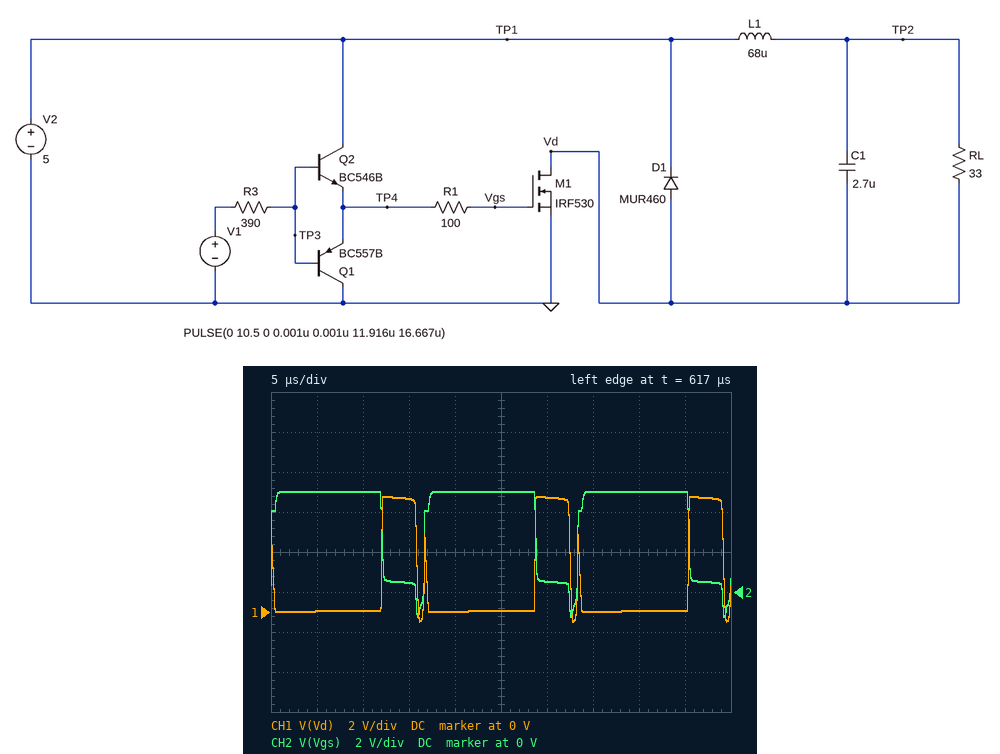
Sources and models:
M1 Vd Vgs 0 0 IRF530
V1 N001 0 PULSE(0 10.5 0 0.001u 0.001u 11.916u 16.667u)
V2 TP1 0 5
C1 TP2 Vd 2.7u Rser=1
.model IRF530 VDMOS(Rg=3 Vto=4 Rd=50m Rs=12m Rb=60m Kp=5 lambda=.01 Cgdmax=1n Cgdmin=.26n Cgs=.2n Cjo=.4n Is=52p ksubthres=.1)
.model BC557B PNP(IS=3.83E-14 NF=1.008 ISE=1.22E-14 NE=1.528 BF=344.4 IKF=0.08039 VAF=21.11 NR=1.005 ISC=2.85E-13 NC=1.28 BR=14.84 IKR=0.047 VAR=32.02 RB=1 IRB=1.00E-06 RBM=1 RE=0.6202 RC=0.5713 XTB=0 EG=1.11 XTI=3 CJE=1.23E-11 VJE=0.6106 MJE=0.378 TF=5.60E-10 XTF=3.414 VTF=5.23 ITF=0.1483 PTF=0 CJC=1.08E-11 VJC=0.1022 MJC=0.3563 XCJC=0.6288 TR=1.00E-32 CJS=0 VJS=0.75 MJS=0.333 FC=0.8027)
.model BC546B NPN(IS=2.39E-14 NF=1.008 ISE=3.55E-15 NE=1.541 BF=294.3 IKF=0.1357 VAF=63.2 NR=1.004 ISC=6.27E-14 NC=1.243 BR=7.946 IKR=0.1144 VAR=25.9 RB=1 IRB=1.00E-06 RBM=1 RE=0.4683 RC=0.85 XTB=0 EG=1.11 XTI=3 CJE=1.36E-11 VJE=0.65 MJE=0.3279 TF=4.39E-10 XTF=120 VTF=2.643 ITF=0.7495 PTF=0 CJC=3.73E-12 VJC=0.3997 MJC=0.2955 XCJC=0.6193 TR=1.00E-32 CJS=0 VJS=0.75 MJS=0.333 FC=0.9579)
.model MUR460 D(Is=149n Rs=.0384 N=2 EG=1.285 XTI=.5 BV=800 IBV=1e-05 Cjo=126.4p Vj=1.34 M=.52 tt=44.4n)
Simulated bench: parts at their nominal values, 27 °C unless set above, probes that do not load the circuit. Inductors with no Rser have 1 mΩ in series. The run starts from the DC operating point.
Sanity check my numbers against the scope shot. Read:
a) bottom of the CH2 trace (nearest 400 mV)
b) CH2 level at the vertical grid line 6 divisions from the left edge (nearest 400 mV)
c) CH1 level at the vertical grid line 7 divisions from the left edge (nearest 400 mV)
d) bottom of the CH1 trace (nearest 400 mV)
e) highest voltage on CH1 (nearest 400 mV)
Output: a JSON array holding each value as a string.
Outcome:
["-1.2 V", "400 mV", "0 V", "-400 mV", "5.6 V"]
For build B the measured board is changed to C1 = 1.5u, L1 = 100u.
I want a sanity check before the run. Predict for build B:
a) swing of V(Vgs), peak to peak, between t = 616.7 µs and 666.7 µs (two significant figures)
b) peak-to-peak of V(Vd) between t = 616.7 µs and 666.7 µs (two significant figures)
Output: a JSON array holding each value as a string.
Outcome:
["4.6 V", "5.7 V"]
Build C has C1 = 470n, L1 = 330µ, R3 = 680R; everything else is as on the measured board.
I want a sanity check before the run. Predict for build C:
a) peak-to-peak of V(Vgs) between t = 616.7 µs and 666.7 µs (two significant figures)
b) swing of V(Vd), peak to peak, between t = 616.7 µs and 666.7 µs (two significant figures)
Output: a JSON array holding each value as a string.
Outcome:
["4.5 V", "5.7 V"]
